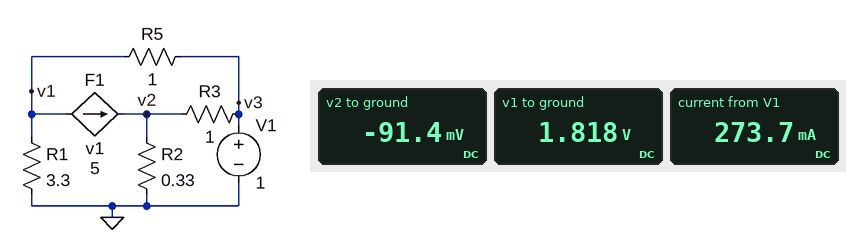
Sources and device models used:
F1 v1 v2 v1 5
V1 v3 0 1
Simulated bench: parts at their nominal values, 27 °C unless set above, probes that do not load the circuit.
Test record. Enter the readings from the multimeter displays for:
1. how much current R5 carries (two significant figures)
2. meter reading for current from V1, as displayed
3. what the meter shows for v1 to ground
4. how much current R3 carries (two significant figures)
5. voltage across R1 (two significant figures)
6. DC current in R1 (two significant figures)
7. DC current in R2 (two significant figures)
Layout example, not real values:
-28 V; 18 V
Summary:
820 mA; 273.7 mA; 1.818 V; 1.1 A; 1.8 V; 550 mA; 280 mA
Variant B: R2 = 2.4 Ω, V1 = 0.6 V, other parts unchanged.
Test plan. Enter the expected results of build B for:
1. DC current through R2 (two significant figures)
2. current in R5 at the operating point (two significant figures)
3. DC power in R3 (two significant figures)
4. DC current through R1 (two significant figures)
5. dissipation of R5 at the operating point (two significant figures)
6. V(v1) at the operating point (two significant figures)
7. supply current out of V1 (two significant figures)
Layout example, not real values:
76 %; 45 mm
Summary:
180 mA; 790 mA; 1.1 W; 420 mA; 620 mW; 1.4 V; 240 mA
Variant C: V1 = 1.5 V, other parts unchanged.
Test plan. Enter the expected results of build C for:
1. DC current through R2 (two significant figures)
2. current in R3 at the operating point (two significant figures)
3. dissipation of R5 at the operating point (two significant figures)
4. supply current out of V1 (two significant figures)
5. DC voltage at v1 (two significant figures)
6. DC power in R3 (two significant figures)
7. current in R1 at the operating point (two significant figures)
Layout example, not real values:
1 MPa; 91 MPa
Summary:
420 mA; 1.6 A; 1.5 W; 410 mA; 2.7 V; 2.7 W; 830 mA
